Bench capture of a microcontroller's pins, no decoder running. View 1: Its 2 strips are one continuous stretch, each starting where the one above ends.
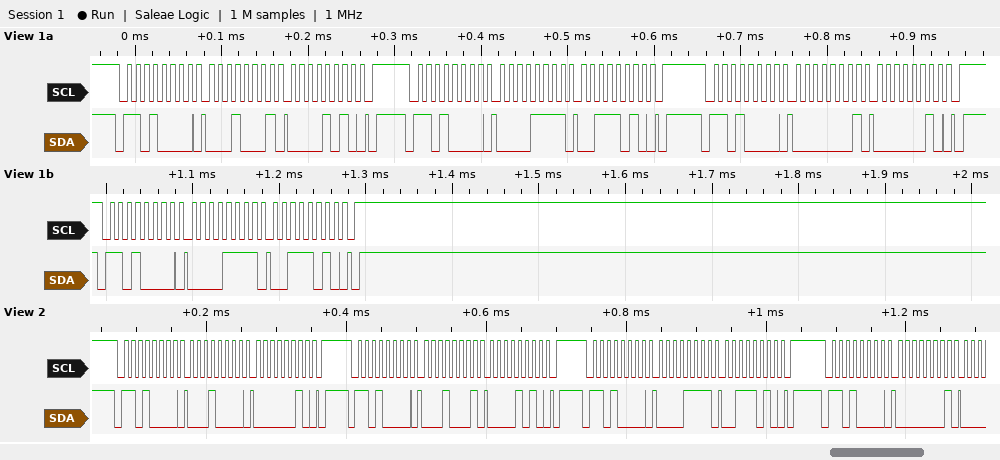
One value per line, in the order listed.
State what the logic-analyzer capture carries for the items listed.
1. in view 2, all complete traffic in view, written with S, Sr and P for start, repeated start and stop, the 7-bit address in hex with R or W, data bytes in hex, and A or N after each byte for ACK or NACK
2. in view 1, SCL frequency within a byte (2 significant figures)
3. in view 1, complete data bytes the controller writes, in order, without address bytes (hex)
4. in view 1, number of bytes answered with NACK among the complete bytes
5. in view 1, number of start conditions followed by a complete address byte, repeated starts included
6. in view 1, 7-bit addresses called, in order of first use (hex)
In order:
S 68W A 10 A 02 A P S 68W A 11 A 0A A P S 68W A 0F A 3A A P S 68W A 01 A
100 kHz
11 0A 0F 3A 01 02 0F 3A
0
4
0x68
